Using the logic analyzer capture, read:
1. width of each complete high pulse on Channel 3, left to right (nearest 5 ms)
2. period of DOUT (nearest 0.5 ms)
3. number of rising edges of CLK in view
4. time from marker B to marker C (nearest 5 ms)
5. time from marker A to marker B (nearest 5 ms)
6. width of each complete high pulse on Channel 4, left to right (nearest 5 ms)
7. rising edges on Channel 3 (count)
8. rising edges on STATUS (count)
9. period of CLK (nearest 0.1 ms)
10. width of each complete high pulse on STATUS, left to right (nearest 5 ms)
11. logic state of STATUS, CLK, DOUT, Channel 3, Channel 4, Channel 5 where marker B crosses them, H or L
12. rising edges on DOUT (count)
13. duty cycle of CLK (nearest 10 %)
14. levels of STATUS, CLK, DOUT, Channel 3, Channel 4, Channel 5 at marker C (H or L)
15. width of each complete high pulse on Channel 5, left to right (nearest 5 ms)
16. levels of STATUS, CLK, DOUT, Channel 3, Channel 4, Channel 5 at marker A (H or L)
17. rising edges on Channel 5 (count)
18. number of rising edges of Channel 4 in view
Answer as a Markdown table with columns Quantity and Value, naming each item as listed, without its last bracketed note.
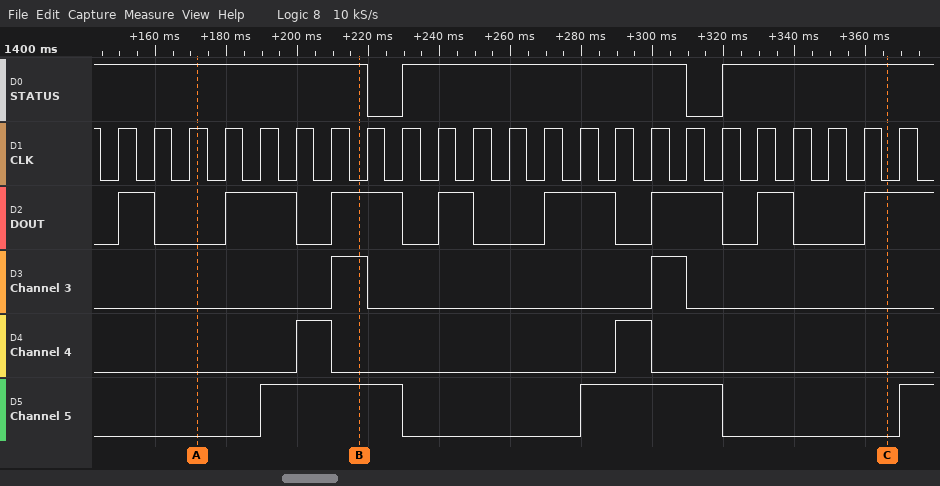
| Quantity | Value |
|---|---|
| width of each complete high pulse on Channel 3, left to right | 10 ms, 10 ms |
| period of DOUT | 30 ms |
| number of rising edges of CLK in view | 23 |
| time from marker B to marker C | 150 ms |
| time from marker A to marker B | 45 ms |
| width of each complete high pulse on Channel 4, left to right | 10 ms, 10 ms |
| rising edges on Channel 3 | 2 |
| rising edges on STATUS | 2 |
| period of CLK | 10 ms |
| width of each complete high pulse on STATUS, left to right | 80 ms |
| logic state of STATUS, CLK, DOUT, Channel 3, Channel 4, Channel 5 where marker B crosses them, H or L | STATUS=H, CLK=L, DOUT=H, Channel 3=H, Channel 4=L, Channel 5=H |
| rising edges on DOUT | 8 |
| duty cycle of CLK | 50 % |
| levels of STATUS, CLK, DOUT, Channel 3, Channel 4, Channel 5 at marker C | STATUS=H, CLK=L, DOUT=H, Channel 3=L, Channel 4=L, Channel 5=L |
| width of each complete high pulse on Channel 5, left to right | 40 ms, 40 ms |
| levels of STATUS, CLK, DOUT, Channel 3, Channel 4, Channel 5 at marker A | STATUS=H, CLK=H, DOUT=L, Channel 3=L, Channel 4=L, Channel 5=L |
| rising edges on Channel 5 | 3 |
| number of rising edges of Channel 4 in view | 2 |
